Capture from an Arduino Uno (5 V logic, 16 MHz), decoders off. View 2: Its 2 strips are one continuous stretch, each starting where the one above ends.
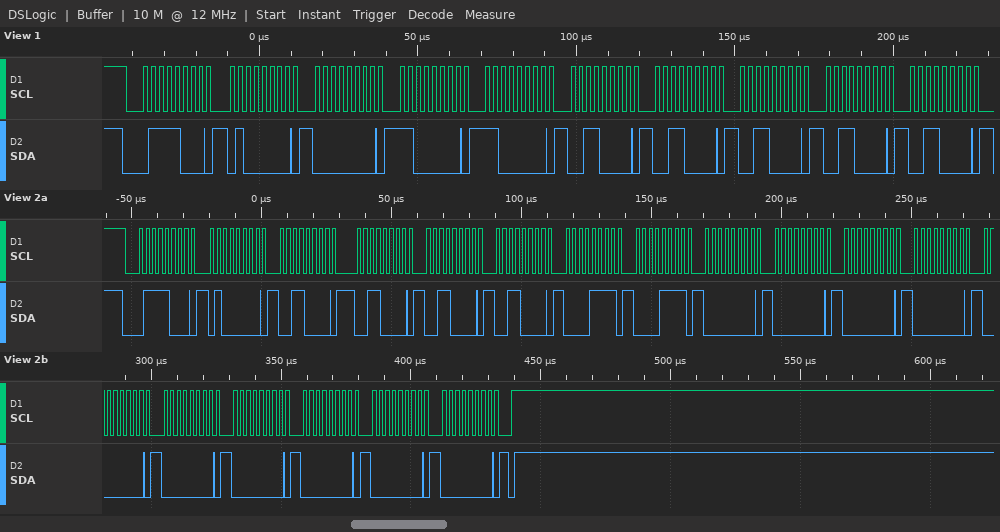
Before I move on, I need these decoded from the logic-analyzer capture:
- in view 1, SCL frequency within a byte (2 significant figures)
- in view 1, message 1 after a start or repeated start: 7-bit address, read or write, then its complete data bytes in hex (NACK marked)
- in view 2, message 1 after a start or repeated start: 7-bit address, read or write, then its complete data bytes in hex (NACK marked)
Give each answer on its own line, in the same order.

400 kHz
0x3C write: 40 00 C0 C0 30 30 30 30 30
0x3C write: 40 30 30 30 30 0F 0F 00 00 00 00 00 00 00 00 00 00
